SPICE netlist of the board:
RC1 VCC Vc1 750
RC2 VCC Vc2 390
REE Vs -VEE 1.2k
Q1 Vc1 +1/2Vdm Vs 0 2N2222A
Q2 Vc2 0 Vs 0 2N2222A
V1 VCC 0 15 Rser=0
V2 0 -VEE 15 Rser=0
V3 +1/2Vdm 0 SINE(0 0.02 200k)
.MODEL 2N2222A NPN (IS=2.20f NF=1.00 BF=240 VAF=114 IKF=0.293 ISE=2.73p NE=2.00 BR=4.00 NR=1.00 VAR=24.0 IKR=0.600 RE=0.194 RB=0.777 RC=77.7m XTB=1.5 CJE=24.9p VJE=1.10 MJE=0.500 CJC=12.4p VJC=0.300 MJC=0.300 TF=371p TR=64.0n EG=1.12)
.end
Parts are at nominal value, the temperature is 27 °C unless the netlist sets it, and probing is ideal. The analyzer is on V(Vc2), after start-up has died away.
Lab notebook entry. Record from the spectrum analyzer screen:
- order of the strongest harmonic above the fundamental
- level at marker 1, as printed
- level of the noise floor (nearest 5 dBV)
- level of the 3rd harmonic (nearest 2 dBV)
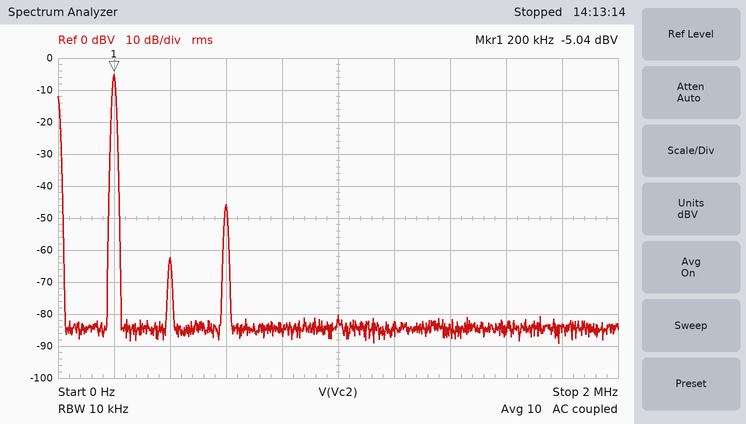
3
-5.04 dBV
-85 dBV
-46 dBV
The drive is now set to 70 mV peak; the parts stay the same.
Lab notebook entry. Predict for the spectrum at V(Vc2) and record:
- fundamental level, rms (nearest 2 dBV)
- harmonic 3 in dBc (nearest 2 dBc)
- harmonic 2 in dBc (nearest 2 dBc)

4 dBV
-20 dBc
-50 dBc
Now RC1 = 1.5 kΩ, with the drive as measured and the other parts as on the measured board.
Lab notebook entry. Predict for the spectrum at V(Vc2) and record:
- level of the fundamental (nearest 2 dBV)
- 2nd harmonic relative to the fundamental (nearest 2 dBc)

-6 dBV
-48 dBc
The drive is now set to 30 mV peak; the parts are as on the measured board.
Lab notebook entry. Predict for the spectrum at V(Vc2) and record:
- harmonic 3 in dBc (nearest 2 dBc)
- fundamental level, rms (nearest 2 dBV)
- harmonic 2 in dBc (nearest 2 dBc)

-34 dBc
-2 dBV
-54 dBc
